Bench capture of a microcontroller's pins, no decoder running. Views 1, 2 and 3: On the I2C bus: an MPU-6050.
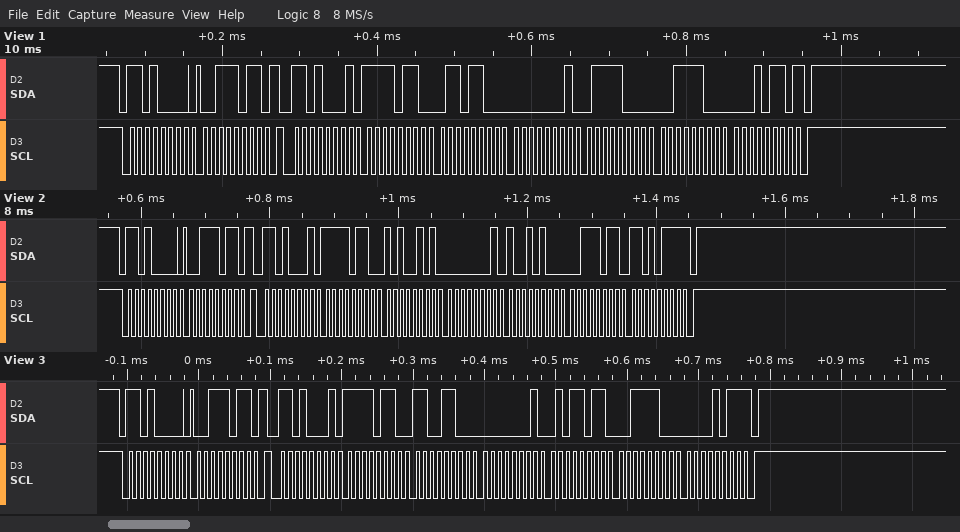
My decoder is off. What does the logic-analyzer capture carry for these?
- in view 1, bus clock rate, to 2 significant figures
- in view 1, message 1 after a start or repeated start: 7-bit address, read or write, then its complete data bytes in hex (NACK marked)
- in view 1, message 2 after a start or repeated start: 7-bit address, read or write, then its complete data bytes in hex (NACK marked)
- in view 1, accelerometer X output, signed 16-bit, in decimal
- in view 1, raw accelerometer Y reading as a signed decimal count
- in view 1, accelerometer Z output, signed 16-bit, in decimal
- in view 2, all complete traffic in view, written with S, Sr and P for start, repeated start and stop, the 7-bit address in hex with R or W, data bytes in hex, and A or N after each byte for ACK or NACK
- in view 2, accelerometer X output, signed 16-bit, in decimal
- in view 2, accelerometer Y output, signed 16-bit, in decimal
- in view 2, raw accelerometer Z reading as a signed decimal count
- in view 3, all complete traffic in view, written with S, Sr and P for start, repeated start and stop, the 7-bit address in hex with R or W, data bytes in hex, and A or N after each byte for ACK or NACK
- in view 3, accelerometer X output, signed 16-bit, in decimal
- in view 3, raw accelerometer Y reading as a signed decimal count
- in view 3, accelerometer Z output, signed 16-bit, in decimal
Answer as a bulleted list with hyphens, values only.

- 100 kHz
- 0x68 write: 3B
- 0x68 read: F6 6C 01 78 3C 16 NACK
- -2452
- 376
- 15382
- S 68W A 3B A Sr 68R A F6 A A5 A 01 A 94 A 3B A D7 N P
- -2395
- 404
- 15319
- S 68W A 3B A Sr 68R A F6 A CC A 01 A 5B A 3C A 0B N P
- -2356
- 347
- 15371
